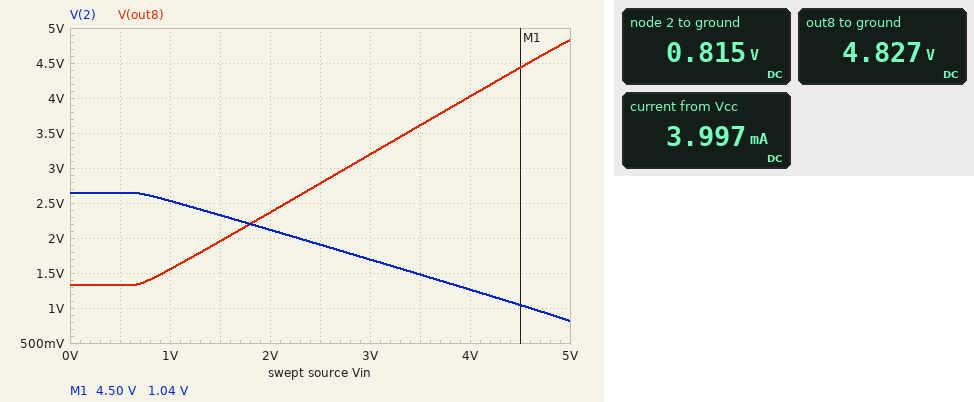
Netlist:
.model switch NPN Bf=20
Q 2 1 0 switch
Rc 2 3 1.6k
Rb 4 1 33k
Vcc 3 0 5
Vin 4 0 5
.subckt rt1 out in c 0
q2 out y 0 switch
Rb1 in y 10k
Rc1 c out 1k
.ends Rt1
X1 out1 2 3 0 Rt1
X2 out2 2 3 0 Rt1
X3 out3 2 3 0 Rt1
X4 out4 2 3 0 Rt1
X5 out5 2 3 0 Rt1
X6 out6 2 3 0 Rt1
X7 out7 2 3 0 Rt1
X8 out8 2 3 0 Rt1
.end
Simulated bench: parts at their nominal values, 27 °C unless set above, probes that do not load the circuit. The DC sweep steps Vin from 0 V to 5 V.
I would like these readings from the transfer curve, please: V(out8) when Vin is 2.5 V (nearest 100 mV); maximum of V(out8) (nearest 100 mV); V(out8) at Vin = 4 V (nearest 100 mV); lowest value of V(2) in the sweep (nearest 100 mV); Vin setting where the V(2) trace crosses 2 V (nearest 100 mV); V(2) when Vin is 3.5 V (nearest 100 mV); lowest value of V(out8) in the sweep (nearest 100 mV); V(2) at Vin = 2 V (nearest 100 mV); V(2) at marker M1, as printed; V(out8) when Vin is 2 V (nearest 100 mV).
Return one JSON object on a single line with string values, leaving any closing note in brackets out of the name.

{"V(out8) when Vin is 2.5 V": "2.8 V", "maximum of V(out8)": "4.8 V", "V(out8) at Vin = 4 V": "4.0 V", "lowest value of V(2) in the sweep": "800 mV", "Vin setting where the V(2) trace crosses 2 V": "2.3 V", "V(2) when Vin is 3.5 V": "1.5 V", "lowest value of V(out8) in the sweep": "1.3 V", "V(2) at Vin = 2 V": "2.1 V", "V(2) at marker M1, as printed": "1.04 V", "V(out8) when Vin is 2 V": "2.4 V"}
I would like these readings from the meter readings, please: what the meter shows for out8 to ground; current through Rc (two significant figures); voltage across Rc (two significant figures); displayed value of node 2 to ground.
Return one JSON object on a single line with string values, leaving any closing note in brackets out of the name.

{"what the meter shows for out8 to ground": "4.827 V", "current through Rc": "2.6 mA", "voltage across Rc": "4.2 V", "displayed value of node 2 to ground": "0.815 V"}
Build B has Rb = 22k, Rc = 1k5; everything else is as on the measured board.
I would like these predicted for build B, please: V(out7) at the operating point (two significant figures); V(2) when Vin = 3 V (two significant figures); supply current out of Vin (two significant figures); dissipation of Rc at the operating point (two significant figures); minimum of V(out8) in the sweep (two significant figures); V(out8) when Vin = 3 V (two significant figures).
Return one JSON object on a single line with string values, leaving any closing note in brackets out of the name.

{"V(out7) at the operating point": "5.0 V", "V(2) when Vin = 3 V": "1.3 V", "supply current out of Vin": "190 µA", "dissipation of Rc at the operating point": "16 mW", "minimum of V(out8) in the sweep": "1.2 V", "V(out8) when Vin = 3 V": "3.9 V"}
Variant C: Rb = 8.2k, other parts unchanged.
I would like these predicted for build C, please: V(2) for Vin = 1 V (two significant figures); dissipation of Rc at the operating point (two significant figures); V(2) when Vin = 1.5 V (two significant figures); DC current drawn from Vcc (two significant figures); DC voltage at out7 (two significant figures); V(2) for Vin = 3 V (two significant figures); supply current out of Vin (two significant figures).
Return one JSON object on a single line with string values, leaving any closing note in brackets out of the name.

{"V(2) for Vin = 1 V": "2.2 V", "dissipation of Rc at the operating point": "15 mW", "V(2) when Vin = 1.5 V": "1.4 V", "DC current drawn from Vcc": "3.1 mA", "DC voltage at out7": "5.0 V", "V(2) for Vin = 3 V": "89 mV", "supply current out of Vin": "510 µA"}
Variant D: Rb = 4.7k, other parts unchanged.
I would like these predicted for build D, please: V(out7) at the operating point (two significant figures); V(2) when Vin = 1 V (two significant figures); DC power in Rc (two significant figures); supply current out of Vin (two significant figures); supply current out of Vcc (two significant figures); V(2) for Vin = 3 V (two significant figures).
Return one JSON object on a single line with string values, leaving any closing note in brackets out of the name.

{"V(out7) at the operating point": "5.0 V", "V(2) when Vin = 1 V": "2.0 V", "DC power in Rc": "15 mW", "supply current out of Vin": "890 µA", "supply current out of Vcc": "3.1 mA", "V(2) for Vin = 3 V": "66 mV"}
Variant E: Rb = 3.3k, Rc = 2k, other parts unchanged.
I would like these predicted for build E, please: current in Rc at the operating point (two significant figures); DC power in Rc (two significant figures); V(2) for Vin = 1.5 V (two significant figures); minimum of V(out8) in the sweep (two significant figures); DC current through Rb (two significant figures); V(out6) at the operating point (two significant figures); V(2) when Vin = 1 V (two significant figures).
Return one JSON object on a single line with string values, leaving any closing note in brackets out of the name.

{"current in Rc at the operating point": "2.5 mA", "DC power in Rc": "12 mW", "V(2) for Vin = 1.5 V": "90 mV", "minimum of V(out8) in the sweep": "1.8 V", "DC current through Rb": "1.3 mA", "V(out6) at the operating point": "5.0 V", "V(2) when Vin = 1 V": "1.4 V"}
